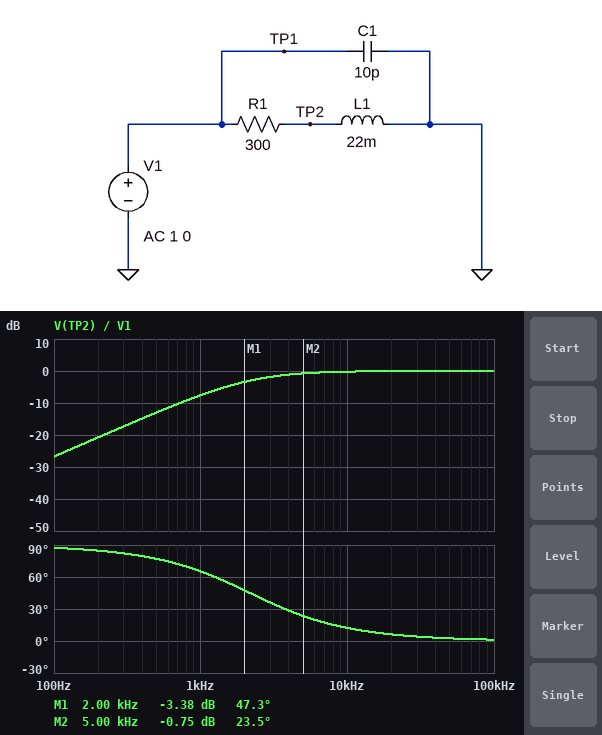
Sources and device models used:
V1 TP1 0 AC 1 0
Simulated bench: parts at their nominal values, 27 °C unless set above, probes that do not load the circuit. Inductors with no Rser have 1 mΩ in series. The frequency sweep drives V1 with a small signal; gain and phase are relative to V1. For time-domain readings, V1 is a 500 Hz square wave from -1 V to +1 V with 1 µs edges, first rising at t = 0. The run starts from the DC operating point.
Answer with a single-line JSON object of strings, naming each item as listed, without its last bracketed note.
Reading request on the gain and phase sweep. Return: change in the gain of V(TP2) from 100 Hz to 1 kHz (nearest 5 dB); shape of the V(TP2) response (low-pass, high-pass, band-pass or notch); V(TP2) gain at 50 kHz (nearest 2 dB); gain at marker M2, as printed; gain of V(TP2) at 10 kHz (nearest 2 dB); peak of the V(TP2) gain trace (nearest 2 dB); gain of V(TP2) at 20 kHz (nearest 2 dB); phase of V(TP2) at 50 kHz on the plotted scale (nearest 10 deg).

{"change in the gain of V(TP2) from 100 Hz to 1 kHz": "20 dB", "shape of the V(TP2) response": "high-pass", "V(TP2) gain at 50 kHz": "0 dB", "gain at marker M2, as printed": "-0.75 dB", "gain of V(TP2) at 10 kHz": "0 dB", "peak of the V(TP2) gain trace": "0 dB", "gain of V(TP2) at 20 kHz": "0 dB", "phase of V(TP2) at 50 kHz on the plotted scale": "0 deg"}
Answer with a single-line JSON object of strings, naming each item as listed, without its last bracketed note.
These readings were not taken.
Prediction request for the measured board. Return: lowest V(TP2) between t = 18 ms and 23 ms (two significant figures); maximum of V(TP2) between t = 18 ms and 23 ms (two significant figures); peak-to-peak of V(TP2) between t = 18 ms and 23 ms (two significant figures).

{"lowest V(TP2) between t = 18 ms and 23 ms": "-2.0 V", "maximum of V(TP2) between t = 18 ms and 23 ms": "2.0 V", "peak-to-peak of V(TP2) between t = 18 ms and 23 ms": "4.0 V"}
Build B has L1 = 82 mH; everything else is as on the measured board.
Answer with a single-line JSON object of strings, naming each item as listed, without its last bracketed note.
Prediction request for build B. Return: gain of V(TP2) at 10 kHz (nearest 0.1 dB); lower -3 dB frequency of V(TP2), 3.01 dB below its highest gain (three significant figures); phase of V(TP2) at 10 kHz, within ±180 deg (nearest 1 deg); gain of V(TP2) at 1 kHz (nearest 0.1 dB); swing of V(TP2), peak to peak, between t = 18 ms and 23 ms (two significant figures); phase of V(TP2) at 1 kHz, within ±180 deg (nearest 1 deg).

{"gain of V(TP2) at 10 kHz": "0 dB", "lower -3 dB frequency of V(TP2), 3.01 dB below its highest gain": "582 Hz", "phase of V(TP2) at 10 kHz, within ±180 deg": "3 deg", "gain of V(TP2) at 1 kHz": "-1.3 dB", "swing of V(TP2), peak to peak, between t = 18 ms and 23 ms": "3.9 V", "phase of V(TP2) at 1 kHz, within ±180 deg": "30 deg"}
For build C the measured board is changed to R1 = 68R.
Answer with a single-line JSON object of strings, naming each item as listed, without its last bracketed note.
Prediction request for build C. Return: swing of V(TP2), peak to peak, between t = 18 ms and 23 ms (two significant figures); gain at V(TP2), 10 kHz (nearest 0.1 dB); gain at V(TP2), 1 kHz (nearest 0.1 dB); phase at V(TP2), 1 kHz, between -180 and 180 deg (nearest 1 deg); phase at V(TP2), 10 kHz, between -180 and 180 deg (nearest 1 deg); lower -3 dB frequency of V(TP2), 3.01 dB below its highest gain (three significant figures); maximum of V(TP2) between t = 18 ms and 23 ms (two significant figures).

{"swing of V(TP2), peak to peak, between t = 18 ms and 23 ms": "3.8 V", "gain at V(TP2), 10 kHz": "0 dB", "gain at V(TP2), 1 kHz": "-0.9 dB", "phase at V(TP2), 1 kHz, between -180 and 180 deg": "26 deg", "phase at V(TP2), 10 kHz, between -180 and 180 deg": "3 deg", "lower -3 dB frequency of V(TP2), 3.01 dB below its highest gain": "492 Hz", "maximum of V(TP2) between t = 18 ms and 23 ms": "1.9 V"}
